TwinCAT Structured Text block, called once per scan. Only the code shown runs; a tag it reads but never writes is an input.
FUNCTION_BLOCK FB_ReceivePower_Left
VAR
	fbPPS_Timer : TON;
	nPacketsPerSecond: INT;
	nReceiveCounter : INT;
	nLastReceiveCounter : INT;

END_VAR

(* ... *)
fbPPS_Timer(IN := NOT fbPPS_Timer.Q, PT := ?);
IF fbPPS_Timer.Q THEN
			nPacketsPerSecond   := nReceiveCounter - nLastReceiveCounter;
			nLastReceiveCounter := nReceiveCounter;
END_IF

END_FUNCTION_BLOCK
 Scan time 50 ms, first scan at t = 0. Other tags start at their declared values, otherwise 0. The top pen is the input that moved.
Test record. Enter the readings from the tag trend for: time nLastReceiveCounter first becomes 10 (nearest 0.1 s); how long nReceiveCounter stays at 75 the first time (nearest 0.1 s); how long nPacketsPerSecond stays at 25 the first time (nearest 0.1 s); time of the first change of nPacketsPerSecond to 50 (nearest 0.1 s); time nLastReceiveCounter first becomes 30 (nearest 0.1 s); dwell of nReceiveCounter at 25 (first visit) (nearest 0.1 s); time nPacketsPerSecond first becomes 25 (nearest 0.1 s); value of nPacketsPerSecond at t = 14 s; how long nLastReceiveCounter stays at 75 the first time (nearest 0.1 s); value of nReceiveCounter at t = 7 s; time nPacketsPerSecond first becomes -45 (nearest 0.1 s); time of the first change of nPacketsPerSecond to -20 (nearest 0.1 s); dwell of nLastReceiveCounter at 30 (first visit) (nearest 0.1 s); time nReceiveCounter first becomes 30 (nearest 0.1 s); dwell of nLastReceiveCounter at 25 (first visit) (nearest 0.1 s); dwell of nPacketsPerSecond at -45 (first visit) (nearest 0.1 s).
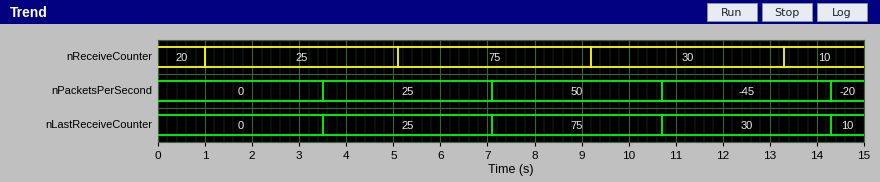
14.3 s
4.1 s
3.6 s
7.1 s
10.7 s
4.1 s
3.5 s
-45
3.6 s
75
10.7 s
14.3 s
3.6 s
9.2 s
3.6 s
3.6 s
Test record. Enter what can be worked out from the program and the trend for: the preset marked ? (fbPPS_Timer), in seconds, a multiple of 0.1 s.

3.5 s
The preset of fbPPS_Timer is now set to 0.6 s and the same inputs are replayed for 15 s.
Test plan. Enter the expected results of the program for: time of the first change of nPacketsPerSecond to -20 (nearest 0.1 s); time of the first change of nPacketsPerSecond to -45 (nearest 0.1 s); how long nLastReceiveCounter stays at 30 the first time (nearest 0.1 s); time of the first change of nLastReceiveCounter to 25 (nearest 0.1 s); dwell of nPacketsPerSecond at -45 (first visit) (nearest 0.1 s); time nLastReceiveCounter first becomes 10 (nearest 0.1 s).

13.9 s
9.7 s
4.2 s
1.3 s
0.7 s
13.9 s
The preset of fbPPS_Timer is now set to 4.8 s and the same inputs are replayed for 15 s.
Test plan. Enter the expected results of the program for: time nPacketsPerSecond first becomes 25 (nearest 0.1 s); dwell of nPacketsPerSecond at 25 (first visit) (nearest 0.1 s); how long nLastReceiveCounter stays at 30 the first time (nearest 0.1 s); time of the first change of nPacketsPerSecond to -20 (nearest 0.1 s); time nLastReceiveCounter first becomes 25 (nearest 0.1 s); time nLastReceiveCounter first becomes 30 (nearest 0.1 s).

4.8 s
4.9 s
4.9 s
14.6 s
4.8 s
9.7 s
